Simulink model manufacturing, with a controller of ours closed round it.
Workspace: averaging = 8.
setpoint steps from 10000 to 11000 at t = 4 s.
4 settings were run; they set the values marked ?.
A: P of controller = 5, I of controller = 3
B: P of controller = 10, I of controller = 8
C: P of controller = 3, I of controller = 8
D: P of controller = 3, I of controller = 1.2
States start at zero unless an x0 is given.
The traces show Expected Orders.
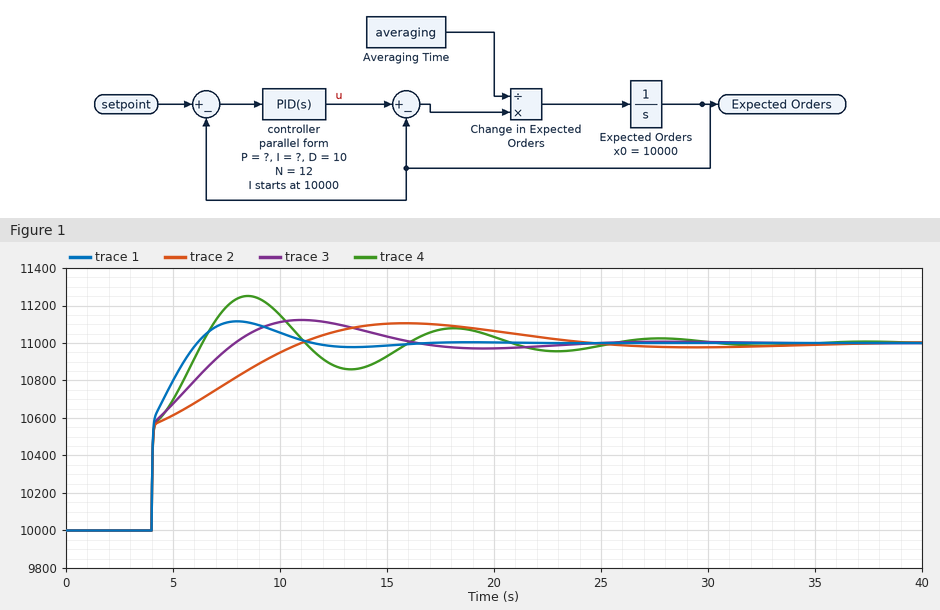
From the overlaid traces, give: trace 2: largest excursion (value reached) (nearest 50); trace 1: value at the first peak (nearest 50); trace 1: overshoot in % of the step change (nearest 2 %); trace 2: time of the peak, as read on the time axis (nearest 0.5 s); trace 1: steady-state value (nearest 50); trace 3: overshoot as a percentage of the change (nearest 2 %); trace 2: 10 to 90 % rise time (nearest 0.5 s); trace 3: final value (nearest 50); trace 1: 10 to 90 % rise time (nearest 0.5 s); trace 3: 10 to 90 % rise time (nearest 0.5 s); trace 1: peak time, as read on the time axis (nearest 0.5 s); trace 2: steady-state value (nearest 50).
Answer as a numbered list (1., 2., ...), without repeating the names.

1. 11100
2. 11100
3. 12 %
4. 16.0 s
5. 11000
6. 12 %
7. 5.0 s
8. 11000
9. 1.5 s
10. 3.0 s
11. 8.0 s
12. 11000
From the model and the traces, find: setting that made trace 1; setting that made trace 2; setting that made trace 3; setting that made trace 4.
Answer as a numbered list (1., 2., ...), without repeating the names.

1. B
2. D
3. A
4. C
